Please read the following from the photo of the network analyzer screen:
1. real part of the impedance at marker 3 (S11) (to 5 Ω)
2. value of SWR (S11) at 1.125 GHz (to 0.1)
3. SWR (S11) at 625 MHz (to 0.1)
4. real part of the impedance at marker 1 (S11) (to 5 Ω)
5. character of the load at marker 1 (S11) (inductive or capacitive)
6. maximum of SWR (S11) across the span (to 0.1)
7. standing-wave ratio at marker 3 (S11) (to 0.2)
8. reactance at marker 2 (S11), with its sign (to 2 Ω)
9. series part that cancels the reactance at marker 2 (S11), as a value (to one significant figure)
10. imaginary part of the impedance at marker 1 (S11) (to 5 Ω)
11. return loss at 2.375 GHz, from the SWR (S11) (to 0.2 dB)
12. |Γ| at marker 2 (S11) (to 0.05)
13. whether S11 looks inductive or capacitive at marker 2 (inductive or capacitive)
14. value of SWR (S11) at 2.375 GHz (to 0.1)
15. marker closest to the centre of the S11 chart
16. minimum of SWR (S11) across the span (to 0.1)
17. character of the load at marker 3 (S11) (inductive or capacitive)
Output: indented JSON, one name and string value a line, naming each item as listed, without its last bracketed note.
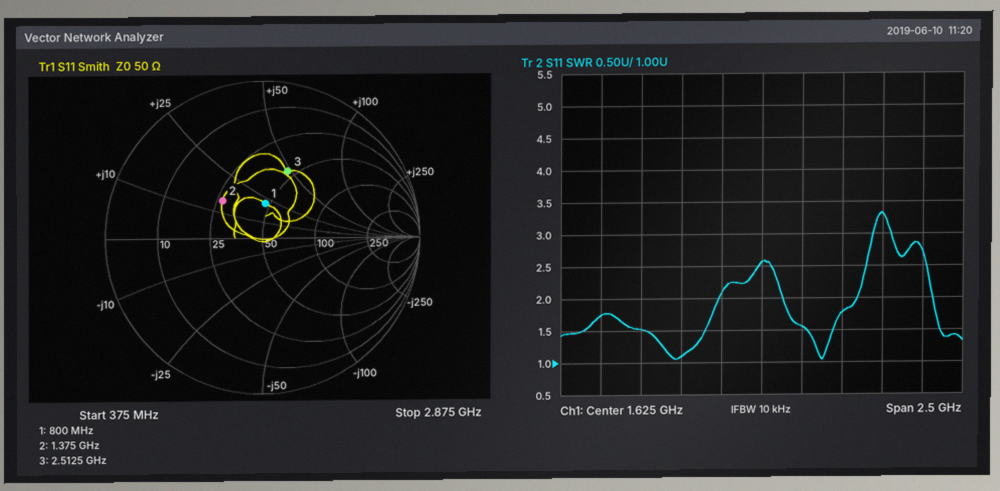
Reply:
{
  "real part of the impedance at marker 3 (S11)": "45 Ω",
  "value of SWR (S11) at 1.125 GHz": "1.1",
  "SWR (S11) at 625 MHz": "1.7",
  "real part of the impedance at marker 1 (S11)": "45 Ω",
  "character of the load at marker 1 (S11)": "inductive",
  "maximum of SWR (S11) across the span": "3.3",
  "standing-wave ratio at marker 3 (S11)": "2.6",
  "reactance at marker 2 (S11), with its sign": "+14 Ω",
  "series part that cancels the reactance at marker 2 (S11), as a value": "8 pF",
  "imaginary part of the impedance at marker 1 (S11)": "+20 Ω",
  "return loss at 2.375 GHz, from the SWR (S11)": "5.4 dB",
  "|Γ| at marker 2 (S11)": "0.35",
  "whether S11 looks inductive or capacitive at marker 2": "inductive",
  "value of SWR (S11) at 2.375 GHz": "3.3",
  "marker closest to the centre of the S11 chart": "marker 1",
  "minimum of SWR (S11) across the span": "1.0",
  "character of the load at marker 3 (S11)": "inductive"
}
